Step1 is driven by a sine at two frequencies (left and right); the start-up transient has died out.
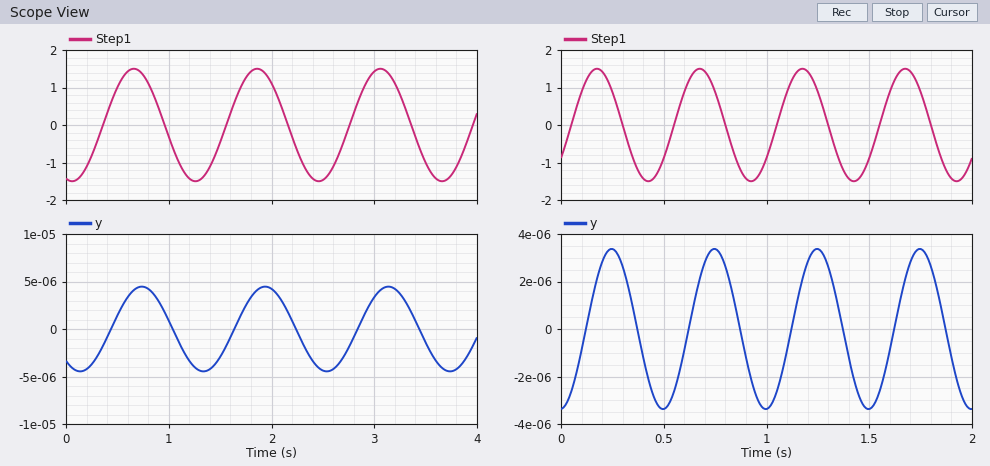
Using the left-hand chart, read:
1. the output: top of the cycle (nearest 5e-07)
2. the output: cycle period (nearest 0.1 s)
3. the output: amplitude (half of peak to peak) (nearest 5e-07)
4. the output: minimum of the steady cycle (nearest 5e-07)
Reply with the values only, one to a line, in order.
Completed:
0.0000045
1.2 s
0.0000045
-0.0000045
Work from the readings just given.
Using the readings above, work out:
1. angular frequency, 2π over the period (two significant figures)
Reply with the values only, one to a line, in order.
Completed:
5.2 rad/s
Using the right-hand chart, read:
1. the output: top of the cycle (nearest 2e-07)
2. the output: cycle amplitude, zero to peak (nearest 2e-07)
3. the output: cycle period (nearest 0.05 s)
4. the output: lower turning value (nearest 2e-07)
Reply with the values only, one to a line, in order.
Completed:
0.0000034
0.0000034
0.50 s
-0.0000034
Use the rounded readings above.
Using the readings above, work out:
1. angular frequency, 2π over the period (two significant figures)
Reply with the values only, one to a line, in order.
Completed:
13 rad/s
